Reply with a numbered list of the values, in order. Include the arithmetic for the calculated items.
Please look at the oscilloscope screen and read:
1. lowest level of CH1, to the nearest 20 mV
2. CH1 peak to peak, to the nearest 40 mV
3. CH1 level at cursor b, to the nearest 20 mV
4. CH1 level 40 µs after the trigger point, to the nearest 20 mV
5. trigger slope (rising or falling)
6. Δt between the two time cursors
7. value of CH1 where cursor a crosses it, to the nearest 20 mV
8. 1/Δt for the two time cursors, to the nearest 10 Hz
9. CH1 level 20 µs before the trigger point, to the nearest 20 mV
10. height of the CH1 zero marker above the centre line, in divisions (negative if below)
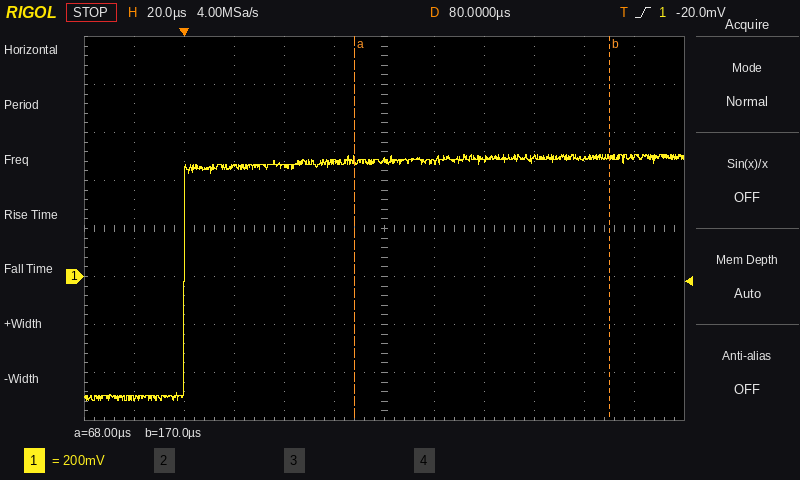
1. -520 mV
2. 1.04 V
3. 500 mV
4. 460 mV
5. rising
6. 170 µs − (68 µs) = 102 µs
7. 480 mV
8. 1 / 102 µs ≈ 9.80 kHz
9. -500 mV
10. -1.0 div
